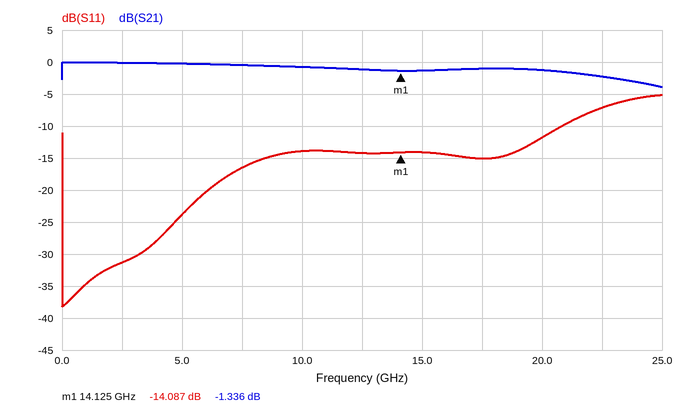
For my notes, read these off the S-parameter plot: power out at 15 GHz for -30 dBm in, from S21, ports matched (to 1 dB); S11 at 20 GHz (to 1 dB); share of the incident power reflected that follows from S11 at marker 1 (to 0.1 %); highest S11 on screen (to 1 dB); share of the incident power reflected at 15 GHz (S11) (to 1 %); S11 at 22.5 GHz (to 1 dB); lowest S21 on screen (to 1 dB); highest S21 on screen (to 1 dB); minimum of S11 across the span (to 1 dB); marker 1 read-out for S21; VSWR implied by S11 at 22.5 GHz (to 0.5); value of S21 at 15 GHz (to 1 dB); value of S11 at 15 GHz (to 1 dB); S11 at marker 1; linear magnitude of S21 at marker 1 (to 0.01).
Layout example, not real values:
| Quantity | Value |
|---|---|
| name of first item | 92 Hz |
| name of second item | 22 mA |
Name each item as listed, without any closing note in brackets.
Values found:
| Quantity | Value |
|---|---|
| power out at 15 GHz for -30 dBm in, from S21, ports matched | -31 dBm |
| S11 at 20 GHz | -12 dB |
| share of the incident power reflected that follows from S11 at marker 1 | 3.9 % |
| highest S11 on screen | -5 dB |
| share of the incident power reflected at 15 GHz (S11) | 4 % |
| S11 at 22.5 GHz | -7 dB |
| lowest S21 on screen | -4 dB |
| highest S21 on screen | 0 dB |
| minimum of S11 across the span | -38 dB |
| marker 1 read-out for S21 | -1.336 dB |
| VSWR implied by S11 at 22.5 GHz | 2.5 |
| value of S21 at 15 GHz | -1 dB |
| value of S11 at 15 GHz | -14 dB |
| S11 at marker 1 | -14.087 dB |
| linear magnitude of S21 at marker 1 | 0.86 |
